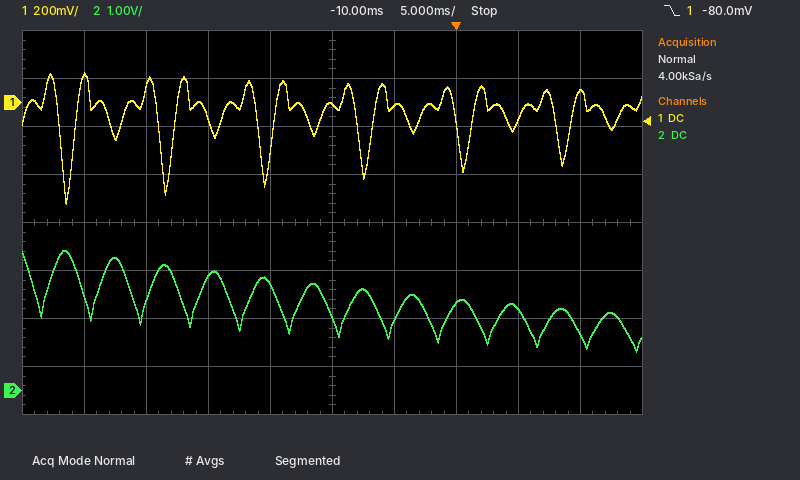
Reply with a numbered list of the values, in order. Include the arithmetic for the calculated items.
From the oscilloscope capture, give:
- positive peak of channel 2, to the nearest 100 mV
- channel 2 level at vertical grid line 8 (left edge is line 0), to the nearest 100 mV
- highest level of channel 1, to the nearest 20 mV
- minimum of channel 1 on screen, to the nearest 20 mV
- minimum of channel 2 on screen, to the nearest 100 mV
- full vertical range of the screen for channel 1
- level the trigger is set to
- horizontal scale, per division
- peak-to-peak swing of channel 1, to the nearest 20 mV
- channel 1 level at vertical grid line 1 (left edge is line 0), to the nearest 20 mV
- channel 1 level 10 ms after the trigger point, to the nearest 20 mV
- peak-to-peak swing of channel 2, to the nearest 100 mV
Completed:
1. 2.9 V
2. 1.7 V
3. 120 mV
4. -420 mV
5. 800 mV
6. 1.6 V
7. -80.0 mV
8. 5 ms
9. 120 mV − (-420 mV) = 540 mV
10. 100 mV
11. 40 mV
12. 2.9 V − (800 mV) = 2.1 V
